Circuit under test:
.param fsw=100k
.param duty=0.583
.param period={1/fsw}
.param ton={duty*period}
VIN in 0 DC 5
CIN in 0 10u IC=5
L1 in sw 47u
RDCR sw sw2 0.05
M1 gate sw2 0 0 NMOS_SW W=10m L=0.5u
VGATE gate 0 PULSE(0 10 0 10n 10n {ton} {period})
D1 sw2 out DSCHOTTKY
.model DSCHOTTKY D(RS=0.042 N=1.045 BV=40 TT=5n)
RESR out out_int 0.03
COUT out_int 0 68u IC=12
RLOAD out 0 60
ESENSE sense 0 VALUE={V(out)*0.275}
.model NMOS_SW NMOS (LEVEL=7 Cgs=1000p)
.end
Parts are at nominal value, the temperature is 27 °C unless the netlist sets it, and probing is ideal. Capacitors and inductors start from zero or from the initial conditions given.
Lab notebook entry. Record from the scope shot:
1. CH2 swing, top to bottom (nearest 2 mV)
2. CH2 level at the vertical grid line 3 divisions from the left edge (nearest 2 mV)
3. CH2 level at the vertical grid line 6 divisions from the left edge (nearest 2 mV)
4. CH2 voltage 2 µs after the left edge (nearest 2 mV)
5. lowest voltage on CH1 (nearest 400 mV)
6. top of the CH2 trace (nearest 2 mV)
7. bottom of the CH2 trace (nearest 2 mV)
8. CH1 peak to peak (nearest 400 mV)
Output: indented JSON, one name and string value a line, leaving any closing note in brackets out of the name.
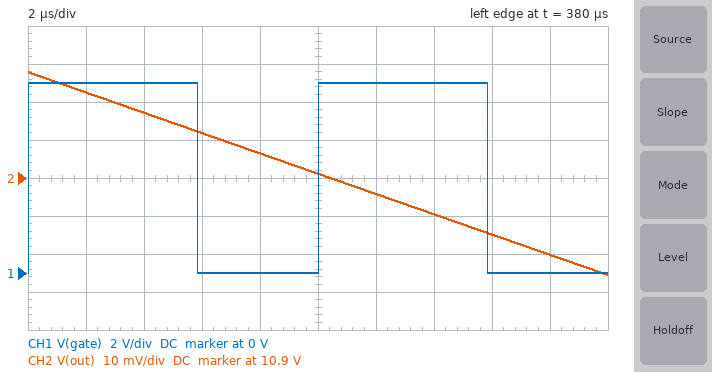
{
  "CH2 swing, top to bottom": "54 mV",
  "CH2 level at the vertical grid line 3 divisions from the left edge": "10.912 V",
  "CH2 level at the vertical grid line 6 divisions from the left edge": "10.896 V",
  "CH2 voltage 2 µs after the left edge": "10.922 V",
  "lowest voltage on CH1": "0 V",
  "top of the CH2 trace": "10.928 V",
  "bottom of the CH2 trace": "10.874 V",
  "CH1 peak to peak": "10.0 V"
}
